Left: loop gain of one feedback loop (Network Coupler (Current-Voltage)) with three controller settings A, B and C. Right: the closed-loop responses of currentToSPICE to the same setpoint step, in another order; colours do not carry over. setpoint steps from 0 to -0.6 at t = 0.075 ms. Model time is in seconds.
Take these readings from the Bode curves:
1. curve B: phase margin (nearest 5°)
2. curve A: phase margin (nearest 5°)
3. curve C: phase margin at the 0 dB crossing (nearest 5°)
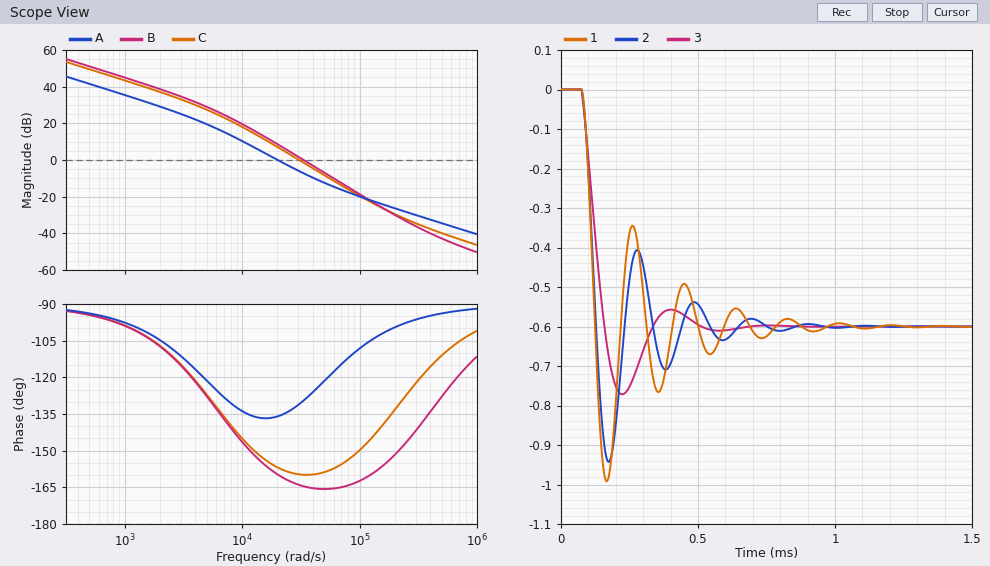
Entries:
15°
45°
20°
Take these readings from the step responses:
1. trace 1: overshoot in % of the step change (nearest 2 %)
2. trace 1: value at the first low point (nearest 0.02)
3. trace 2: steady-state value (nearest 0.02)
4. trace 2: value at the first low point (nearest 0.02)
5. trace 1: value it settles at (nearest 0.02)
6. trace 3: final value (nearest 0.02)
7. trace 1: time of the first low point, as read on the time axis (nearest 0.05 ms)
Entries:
66 %
-1.00
-0.60
-0.94
-0.60
-0.60
0.15 ms
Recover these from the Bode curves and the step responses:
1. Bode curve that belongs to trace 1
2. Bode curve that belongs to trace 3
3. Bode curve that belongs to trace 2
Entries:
B
A
C
